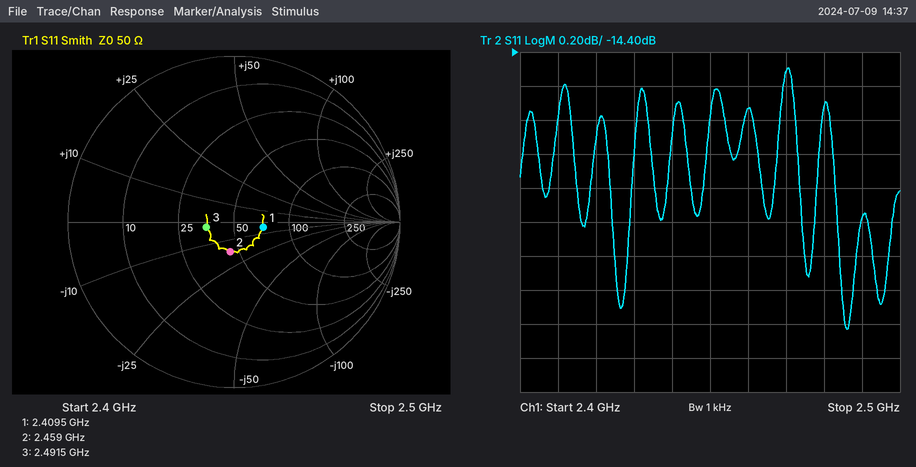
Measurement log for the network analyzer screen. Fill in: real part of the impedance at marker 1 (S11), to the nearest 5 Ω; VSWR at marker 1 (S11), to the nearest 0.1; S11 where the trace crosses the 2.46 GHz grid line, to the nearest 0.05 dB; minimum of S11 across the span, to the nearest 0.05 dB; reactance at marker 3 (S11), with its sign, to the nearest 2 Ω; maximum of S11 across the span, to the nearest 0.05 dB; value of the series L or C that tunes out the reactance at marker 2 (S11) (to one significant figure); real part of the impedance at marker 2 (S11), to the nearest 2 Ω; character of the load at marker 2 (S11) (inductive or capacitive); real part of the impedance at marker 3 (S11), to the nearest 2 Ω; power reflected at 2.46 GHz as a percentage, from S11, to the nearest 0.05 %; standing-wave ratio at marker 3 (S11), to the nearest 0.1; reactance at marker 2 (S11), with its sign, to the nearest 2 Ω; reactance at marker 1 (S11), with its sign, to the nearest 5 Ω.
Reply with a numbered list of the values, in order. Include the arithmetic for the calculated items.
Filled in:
1. 70 Ω
2. 1.4
3. -14.75 dB
4. -16.05 dB
5. -2 Ω
6. -14.50 dB
7. L = 16 Ω/(2π × 2.459 GHz) ≈ 1 nH
8. 44 Ω
9. capacitive
10. 36 Ω
11. 10^(-14.75/10) ≈ 3.35 %
12. 1.4
13. -16 Ω
14. -5 Ω
